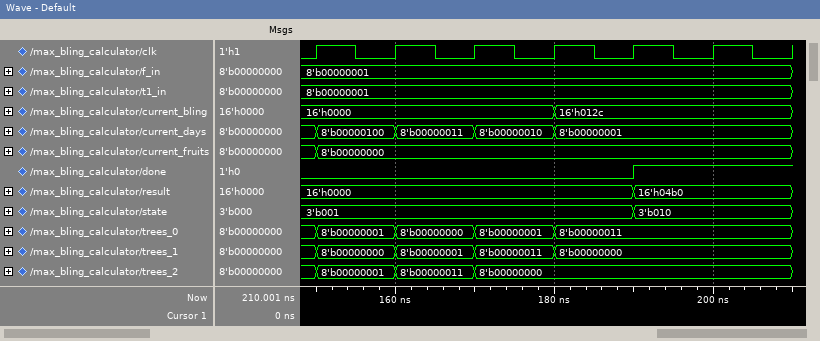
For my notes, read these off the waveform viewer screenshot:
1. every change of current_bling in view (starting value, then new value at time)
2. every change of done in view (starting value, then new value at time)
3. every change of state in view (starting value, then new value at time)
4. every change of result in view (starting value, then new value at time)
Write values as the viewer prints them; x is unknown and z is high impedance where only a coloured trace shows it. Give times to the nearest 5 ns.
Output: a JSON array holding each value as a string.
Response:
["16'h0000, 16'h012c at 180 ns", "0, 1 at 190 ns", "3'b001, 3'b010 at 190 ns", "16'h0000, 16'h04b0 at 190 ns"]
